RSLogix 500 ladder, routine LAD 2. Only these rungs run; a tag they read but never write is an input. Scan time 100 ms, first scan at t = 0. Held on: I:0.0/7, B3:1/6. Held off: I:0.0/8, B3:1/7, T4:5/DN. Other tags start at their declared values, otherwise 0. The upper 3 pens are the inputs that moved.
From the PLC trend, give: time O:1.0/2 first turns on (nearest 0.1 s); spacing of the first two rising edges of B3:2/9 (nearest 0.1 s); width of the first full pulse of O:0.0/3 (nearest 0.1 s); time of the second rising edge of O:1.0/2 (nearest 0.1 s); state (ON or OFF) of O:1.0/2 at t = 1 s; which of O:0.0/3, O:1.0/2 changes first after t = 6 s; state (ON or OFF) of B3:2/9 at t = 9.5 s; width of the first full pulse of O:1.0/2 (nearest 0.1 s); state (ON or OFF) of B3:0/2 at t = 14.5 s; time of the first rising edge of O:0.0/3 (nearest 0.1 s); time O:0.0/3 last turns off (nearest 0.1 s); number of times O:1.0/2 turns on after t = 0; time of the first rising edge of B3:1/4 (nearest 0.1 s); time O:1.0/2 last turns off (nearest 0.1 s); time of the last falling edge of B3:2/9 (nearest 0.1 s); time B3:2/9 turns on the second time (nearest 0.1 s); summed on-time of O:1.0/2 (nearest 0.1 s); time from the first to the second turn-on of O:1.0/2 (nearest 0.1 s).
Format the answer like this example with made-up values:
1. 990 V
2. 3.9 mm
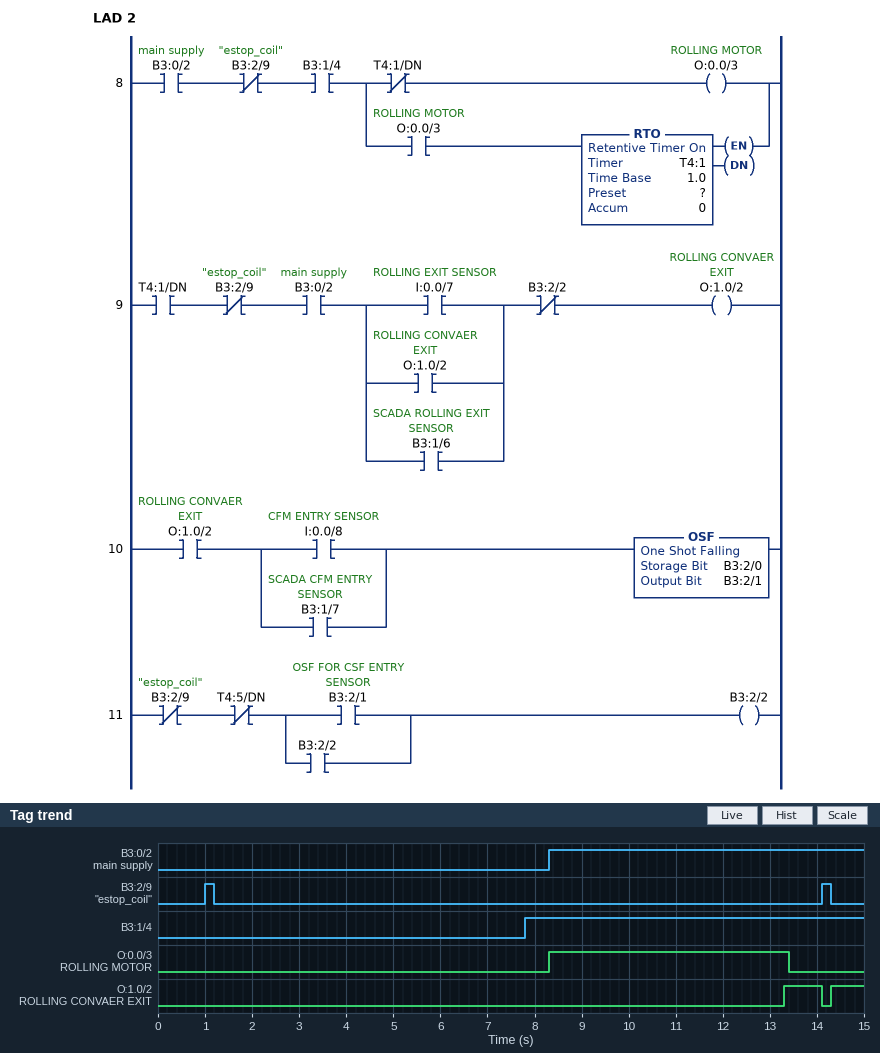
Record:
1. 13.3 s
2. 13.1 s
3. 5.1 s
4. 14.3 s
5. OFF
6. O:0.0/3
7. OFF
8. 0.8 s
9. ON
10. 8.3 s
11. 13.4 s
12. 2
13. 7.8 s
14. 14.1 s
15. 14.3 s
16. 14.1 s
17. 1.5 s
18. 1.0 s
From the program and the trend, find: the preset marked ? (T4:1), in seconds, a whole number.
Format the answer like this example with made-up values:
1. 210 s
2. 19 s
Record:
1. 5 s
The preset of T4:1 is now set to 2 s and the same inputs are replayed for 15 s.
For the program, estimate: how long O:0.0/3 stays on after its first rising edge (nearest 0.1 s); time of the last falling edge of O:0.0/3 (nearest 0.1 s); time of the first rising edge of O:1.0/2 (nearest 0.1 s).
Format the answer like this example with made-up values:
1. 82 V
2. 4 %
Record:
1. 2.1 s
2. 10.4 s
3. 10.3 s
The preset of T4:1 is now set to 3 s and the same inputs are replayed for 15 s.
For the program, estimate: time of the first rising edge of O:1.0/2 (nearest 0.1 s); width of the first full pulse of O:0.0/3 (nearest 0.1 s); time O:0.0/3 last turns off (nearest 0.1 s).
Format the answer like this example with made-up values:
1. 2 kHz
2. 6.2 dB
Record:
1. 11.3 s
2. 3.1 s
3. 11.4 s
